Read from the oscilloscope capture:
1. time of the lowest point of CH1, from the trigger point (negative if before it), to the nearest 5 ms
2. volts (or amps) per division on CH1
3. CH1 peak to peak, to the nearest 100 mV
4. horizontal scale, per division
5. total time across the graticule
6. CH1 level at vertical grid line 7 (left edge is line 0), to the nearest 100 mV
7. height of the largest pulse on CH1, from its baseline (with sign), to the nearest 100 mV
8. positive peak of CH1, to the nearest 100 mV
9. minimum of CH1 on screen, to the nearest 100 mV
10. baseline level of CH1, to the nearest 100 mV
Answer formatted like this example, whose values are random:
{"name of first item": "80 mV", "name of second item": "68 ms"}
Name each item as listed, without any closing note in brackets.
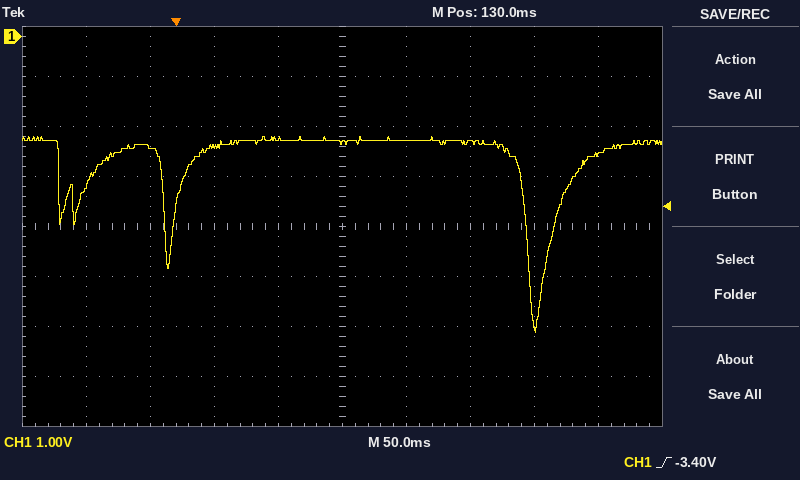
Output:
{"time of the lowest point of CH1, from the trigger point (negative if before it), to the nearest 5 ms": "+280 ms", "volts (or amps) per division on CH1": "1 V", "CH1 peak to peak, to the nearest 100 mV": "3.9 V", "horizontal scale, per division": "50 ms", "total time across the graticule": "500 ms", "CH1 level at vertical grid line 7 (left edge is line 0), to the nearest 100 mV": "-2.1 V", "height of the largest pulse on CH1, from its baseline (with sign), to the nearest 100 mV": "-3.8 V", "positive peak of CH1, to the nearest 100 mV": "-2.0 V", "minimum of CH1 on screen, to the nearest 100 mV": "-5.9 V", "baseline level of CH1, to the nearest 100 mV": "-2.1 V"}
